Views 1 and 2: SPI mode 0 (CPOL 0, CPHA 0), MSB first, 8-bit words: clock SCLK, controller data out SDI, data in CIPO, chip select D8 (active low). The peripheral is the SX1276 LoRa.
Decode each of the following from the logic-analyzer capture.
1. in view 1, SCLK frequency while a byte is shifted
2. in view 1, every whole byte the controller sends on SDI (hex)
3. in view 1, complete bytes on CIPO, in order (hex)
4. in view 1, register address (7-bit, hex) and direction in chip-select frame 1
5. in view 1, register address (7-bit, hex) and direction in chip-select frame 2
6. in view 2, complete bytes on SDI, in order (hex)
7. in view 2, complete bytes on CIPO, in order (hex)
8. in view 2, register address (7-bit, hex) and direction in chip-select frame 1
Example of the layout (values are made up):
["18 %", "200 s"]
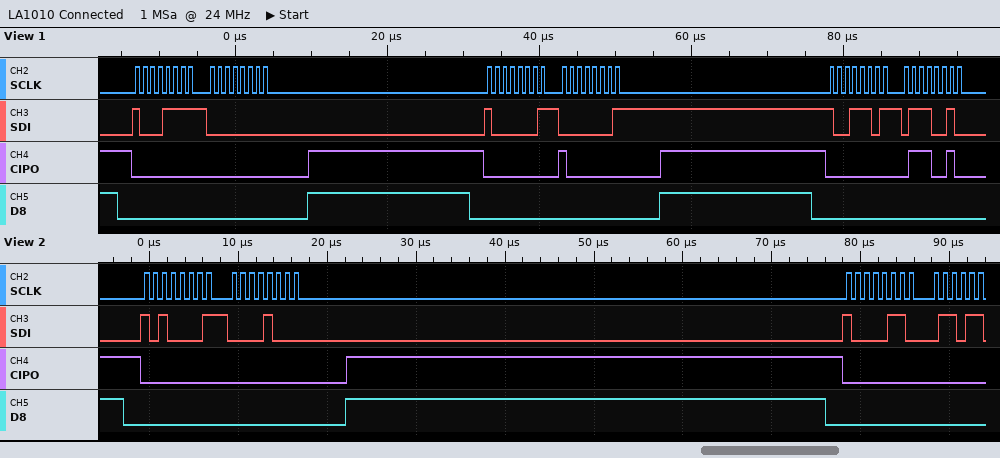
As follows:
["1 MHz", "8F 00 81 01 9D 72", "00 00 00 80 00 72", "0x0F write", "0x01 write", "0xA1 0x08 0x86", "0x00 0x00 0x00", "0x21 write"]
